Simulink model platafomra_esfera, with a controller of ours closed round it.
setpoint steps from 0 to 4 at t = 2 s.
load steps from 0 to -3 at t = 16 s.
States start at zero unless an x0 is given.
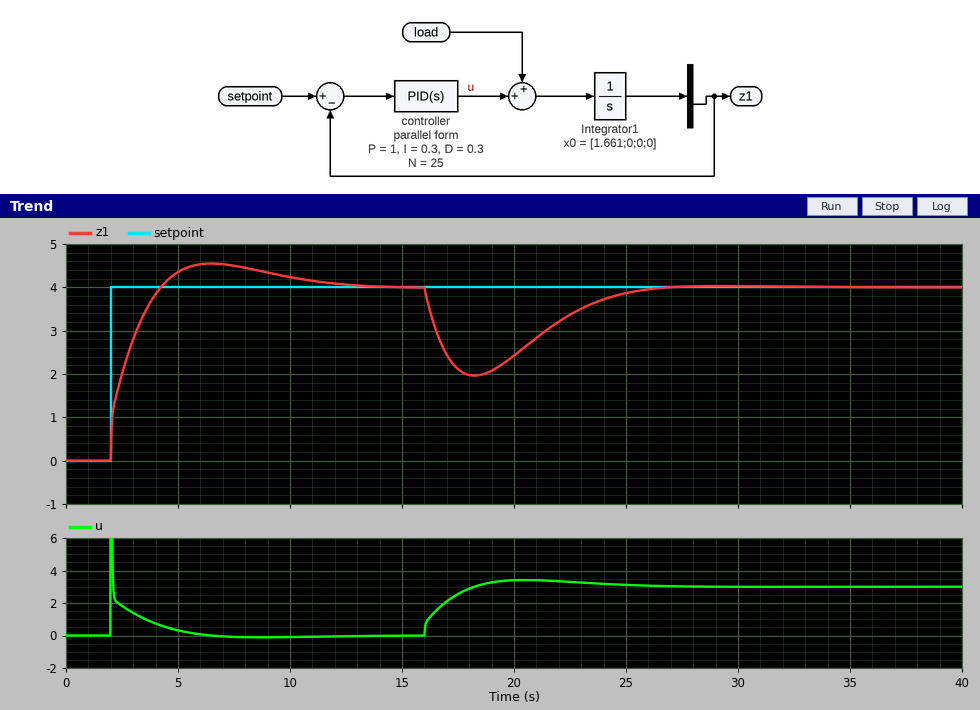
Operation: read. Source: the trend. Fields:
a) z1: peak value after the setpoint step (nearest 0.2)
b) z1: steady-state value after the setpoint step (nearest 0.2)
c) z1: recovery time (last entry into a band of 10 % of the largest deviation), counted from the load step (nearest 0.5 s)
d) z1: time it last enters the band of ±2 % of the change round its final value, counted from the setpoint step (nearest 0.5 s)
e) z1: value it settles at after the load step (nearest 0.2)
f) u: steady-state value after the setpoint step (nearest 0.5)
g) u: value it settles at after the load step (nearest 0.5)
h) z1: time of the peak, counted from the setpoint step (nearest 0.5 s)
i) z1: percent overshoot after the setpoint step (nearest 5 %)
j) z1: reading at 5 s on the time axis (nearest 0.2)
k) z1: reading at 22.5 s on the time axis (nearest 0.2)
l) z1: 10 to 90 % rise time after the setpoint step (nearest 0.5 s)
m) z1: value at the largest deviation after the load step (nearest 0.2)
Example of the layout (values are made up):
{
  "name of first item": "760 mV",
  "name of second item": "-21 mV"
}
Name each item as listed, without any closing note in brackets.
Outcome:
{
  "z1: peak value after the setpoint step": "4.6",
  "z1: steady-state value after the setpoint step": "4.0",
  "z1: recovery time (last entry into a band of 10 % of the largest deviation), counted from the load step": "8.5 s",
  "z1: time it last enters the band of ±2 % of the change round its final value, counted from the setpoint step": "10.0 s",
  "z1: value it settles at after the load step": "4.0",
  "u: steady-state value after the setpoint step": "0.0",
  "u: value it settles at after the load step": "3.0",
  "z1: time of the peak, counted from the setpoint step": "4.5 s",
  "z1: percent overshoot after the setpoint step": "15 %",
  "z1: reading at 5 s on the time axis": "4.4",
  "z1: reading at 22.5 s on the time axis": "3.4",
  "z1: 10 to 90 % rise time after the setpoint step": "1.5 s",
  "z1: value at the largest deviation after the load step": "2.0"
}
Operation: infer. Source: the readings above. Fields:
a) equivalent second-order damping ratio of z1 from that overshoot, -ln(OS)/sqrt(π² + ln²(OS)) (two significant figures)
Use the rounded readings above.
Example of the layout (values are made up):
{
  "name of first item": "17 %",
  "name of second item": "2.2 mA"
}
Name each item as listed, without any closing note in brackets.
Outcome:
{
  "equivalent second-order damping ratio of z1 from that overshoot, -ln(OS)/sqrt(π² + ln²(OS))": "0.52"
}
